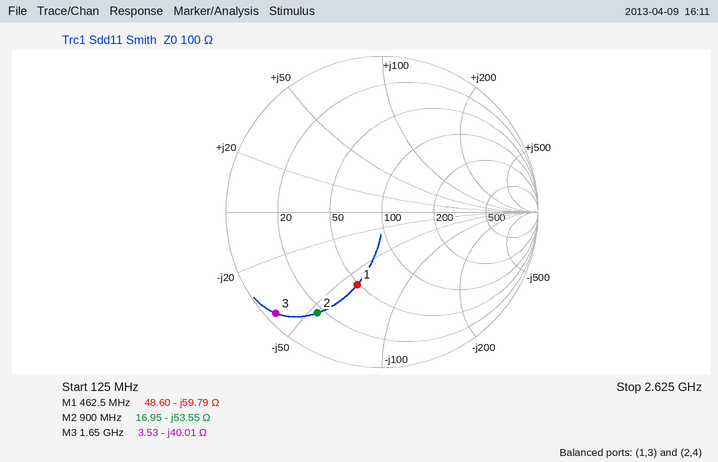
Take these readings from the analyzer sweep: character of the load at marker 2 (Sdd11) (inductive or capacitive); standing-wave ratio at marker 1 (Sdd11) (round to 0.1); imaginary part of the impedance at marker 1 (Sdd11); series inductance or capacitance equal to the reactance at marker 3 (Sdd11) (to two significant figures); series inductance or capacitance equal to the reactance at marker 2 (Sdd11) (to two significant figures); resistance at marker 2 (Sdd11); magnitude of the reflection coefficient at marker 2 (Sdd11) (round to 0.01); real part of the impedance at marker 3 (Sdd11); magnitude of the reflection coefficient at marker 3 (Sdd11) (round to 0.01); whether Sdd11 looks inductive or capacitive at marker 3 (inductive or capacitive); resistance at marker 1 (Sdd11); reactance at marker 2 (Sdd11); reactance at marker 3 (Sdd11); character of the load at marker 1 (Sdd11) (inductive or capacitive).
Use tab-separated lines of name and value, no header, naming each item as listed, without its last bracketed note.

character of the load at marker 2 (Sdd11)	capacitive
standing-wave ratio at marker 1 (Sdd11)	2.9
imaginary part of the impedance at marker 1	-59.79 Ω
series inductance or capacitance equal to the reactance at marker 3 (Sdd11)	2.4 pF
series inductance or capacitance equal to the reactance at marker 2 (Sdd11)	3.3 pF
resistance at marker 2	16.95 Ω
magnitude of the reflection coefficient at marker 2 (Sdd11)	0.77
real part of the impedance at marker 3	3.53 Ω
magnitude of the reflection coefficient at marker 3 (Sdd11)	0.94
whether Sdd11 looks inductive or capacitive at marker 3	capacitive
resistance at marker 1	48.60 Ω
reactance at marker 2	-53.55 Ω
reactance at marker 3	-40.01 Ω
character of the load at marker 1 (Sdd11)	capacitive
